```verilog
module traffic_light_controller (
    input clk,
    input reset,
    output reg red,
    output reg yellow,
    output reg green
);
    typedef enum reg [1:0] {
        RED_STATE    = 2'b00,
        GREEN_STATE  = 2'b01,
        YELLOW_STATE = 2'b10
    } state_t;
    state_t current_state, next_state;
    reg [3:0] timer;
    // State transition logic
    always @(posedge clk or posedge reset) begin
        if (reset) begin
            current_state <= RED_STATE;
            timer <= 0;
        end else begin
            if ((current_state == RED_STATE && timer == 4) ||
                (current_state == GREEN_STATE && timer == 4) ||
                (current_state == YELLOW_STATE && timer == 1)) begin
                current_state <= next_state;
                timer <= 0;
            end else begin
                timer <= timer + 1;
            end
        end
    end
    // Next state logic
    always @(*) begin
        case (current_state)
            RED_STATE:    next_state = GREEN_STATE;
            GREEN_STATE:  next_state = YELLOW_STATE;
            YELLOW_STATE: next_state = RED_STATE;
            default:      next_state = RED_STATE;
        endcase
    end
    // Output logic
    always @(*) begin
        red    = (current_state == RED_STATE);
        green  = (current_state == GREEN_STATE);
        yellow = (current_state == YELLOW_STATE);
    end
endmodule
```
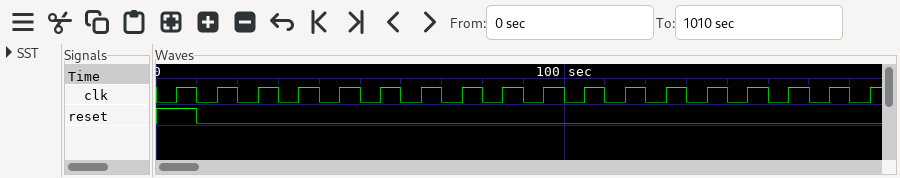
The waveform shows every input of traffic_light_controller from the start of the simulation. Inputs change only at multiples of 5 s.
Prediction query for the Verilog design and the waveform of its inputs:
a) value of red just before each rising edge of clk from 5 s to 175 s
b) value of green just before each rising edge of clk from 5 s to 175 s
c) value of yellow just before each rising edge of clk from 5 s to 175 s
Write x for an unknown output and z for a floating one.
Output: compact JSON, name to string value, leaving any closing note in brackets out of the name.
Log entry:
{"value of red just before each rising edge of clk from 5 s to 175 s": "1 1 1 1 1 1 0 0 0 0 0 0 0 1 1 1 1 1", "value of green just before each rising edge of clk from 5 s to 175 s": "0 0 0 0 0 0 1 1 1 1 1 0 0 0 0 0 0 0", "value of yellow just before each rising edge of clk from 5 s to 175 s": "0 0 0 0 0 0 0 0 0 0 0 1 1 0 0 0 0 0"}
